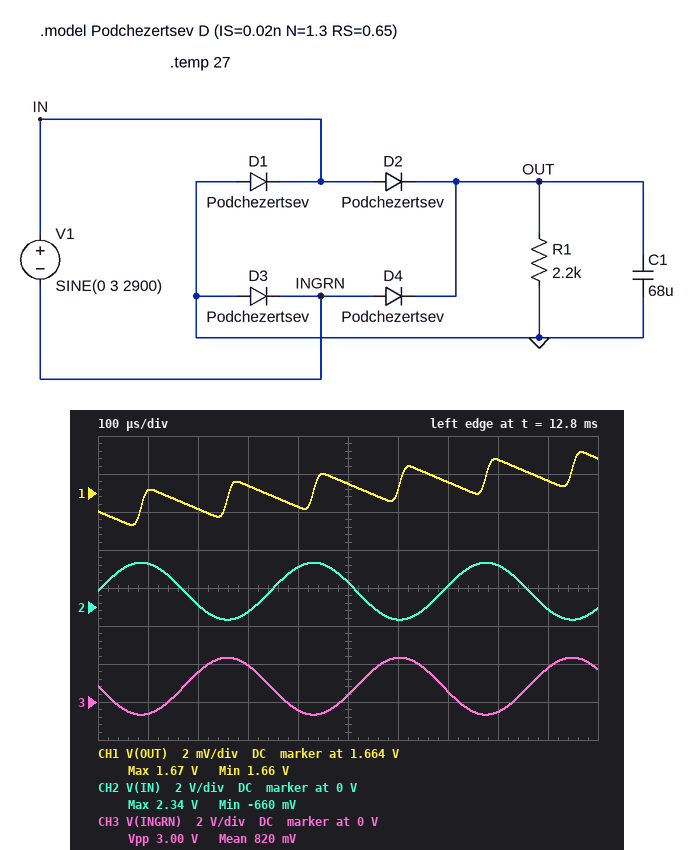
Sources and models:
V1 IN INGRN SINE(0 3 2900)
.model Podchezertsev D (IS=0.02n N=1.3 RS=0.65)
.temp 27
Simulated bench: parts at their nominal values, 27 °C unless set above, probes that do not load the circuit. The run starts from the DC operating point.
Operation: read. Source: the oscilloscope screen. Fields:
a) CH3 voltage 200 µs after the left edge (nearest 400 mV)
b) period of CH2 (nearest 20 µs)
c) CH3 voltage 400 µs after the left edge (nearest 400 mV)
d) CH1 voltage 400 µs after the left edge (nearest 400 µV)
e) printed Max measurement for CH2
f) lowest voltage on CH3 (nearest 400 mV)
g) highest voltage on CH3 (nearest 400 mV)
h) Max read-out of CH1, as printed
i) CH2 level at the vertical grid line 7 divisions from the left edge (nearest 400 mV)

1.6 V
340 µs
-400 mV
1.6632 V
2.34 V
-800 mV
2.4 V
1.67 V
1.2 V
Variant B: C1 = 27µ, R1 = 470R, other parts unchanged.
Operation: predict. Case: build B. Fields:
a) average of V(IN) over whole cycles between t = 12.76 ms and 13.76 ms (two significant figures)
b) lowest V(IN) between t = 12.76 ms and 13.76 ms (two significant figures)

780 mV
-720 mV
